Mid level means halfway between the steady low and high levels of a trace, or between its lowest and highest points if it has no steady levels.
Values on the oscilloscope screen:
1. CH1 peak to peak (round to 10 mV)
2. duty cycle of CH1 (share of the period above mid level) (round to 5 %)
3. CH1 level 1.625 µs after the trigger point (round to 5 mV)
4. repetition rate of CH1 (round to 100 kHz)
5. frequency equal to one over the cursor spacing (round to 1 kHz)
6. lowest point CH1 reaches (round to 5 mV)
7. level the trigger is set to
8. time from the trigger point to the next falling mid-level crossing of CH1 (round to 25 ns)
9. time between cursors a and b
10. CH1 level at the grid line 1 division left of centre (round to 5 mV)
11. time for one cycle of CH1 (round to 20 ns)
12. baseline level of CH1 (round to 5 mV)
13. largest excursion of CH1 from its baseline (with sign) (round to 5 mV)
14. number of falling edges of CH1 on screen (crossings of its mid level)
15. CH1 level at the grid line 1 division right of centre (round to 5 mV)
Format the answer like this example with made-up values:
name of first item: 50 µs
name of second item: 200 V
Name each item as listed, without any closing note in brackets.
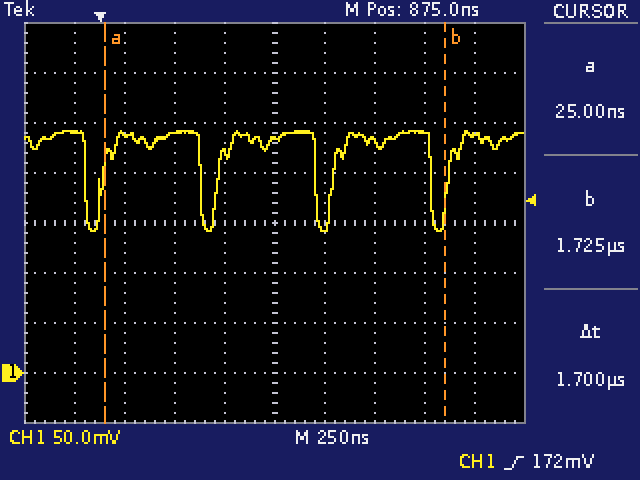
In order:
CH1 peak to peak: 100 mV
duty cycle of CH1 (share of the period above mid level): 85 %
CH1 level 1.625 µs after the trigger point: 240 mV
repetition rate of CH1: 1.7 MHz
frequency equal to one over the cursor spacing: 588 kHz
lowest point CH1 reaches: 140 mV
level the trigger is set to: 172 mV
time from the trigger point to the next falling mid-level crossing of CH1: 500 ns
time between cursors a and b: 1.7 µs
CH1 level at the grid line 1 division left of centre: 220 mV
time for one cycle of CH1: 580 ns
baseline level of CH1: 235 mV
largest excursion of CH1 from its baseline (with sign): -95 mV
number of falling edges of CH1 on screen: 4
CH1 level at the grid line 1 division right of centre: 145 mV
